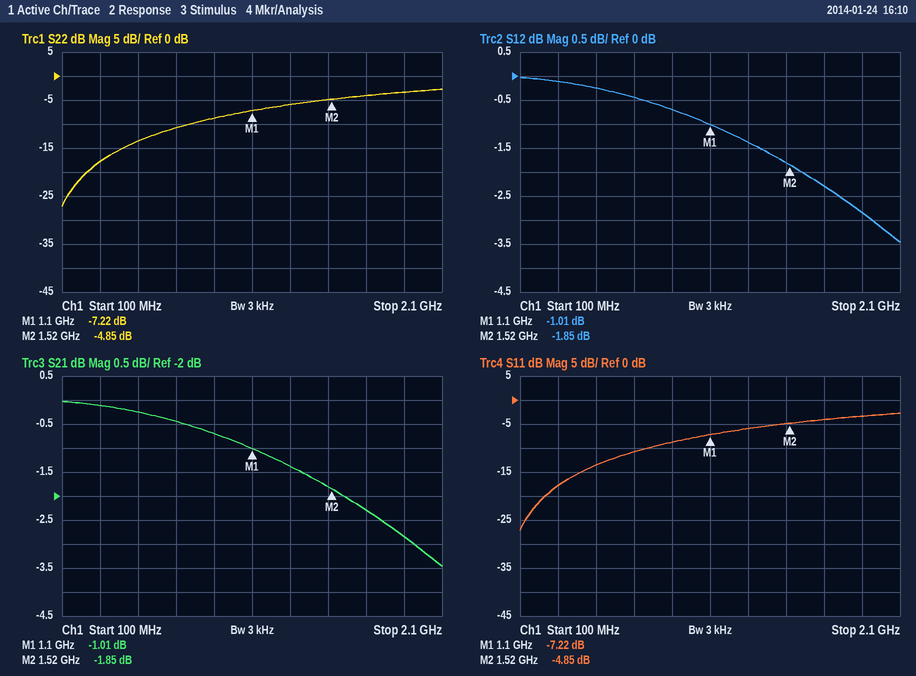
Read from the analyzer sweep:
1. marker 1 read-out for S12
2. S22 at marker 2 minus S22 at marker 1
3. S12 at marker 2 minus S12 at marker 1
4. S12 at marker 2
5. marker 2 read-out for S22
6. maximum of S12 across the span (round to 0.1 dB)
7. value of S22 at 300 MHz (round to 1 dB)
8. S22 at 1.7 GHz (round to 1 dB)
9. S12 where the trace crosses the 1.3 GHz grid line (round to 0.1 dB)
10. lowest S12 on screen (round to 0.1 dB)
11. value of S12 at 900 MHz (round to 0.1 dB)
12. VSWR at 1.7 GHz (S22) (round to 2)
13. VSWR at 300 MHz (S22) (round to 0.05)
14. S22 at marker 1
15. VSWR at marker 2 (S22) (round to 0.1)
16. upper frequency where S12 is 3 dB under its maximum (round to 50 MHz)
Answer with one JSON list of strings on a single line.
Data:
["-1.01 dB", "2.37 dB", "-0.84 dB", "-1.85 dB", "-4.85 dB", "0.0 dB", "-18 dB", "-4 dB", "-1.4 dB", "-3.5 dB", "-0.7 dB", "4", "1.30", "-7.22 dB", "3.7", "1.95 GHz"]
